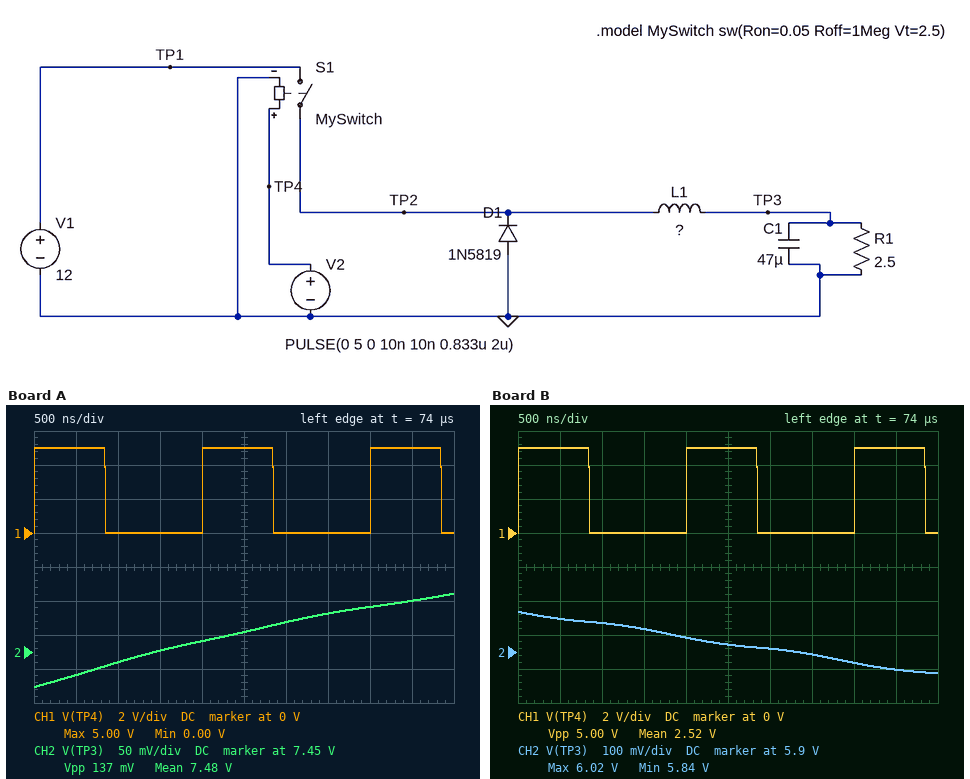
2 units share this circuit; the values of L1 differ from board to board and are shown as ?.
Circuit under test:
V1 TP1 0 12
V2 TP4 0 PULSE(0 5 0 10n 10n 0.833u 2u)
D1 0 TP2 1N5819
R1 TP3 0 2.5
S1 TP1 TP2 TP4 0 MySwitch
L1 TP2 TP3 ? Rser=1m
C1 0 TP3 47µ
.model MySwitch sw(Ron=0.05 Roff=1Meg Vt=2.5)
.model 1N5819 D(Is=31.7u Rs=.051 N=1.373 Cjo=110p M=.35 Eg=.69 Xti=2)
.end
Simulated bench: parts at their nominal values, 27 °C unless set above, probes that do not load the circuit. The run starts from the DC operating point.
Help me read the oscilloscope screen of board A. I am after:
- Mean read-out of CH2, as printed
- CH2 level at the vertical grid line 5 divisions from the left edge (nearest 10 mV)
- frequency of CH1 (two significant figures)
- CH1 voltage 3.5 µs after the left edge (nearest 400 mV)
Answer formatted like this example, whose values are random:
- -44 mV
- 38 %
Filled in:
- 7.48 V
- 7.48 V
- 500 kHz
- 0 V
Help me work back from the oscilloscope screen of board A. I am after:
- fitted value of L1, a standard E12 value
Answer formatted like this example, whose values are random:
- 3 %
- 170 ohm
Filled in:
- 15 µH
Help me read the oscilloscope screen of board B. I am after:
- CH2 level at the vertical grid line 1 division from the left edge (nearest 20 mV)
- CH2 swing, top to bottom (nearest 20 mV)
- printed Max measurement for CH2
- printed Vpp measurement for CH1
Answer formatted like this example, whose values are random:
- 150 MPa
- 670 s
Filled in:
- 6.00 V
- 180 mV
- 6.02 V
- 5.00 V
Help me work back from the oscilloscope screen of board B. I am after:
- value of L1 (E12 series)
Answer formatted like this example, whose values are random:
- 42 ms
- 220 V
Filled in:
- 3.3 µH
